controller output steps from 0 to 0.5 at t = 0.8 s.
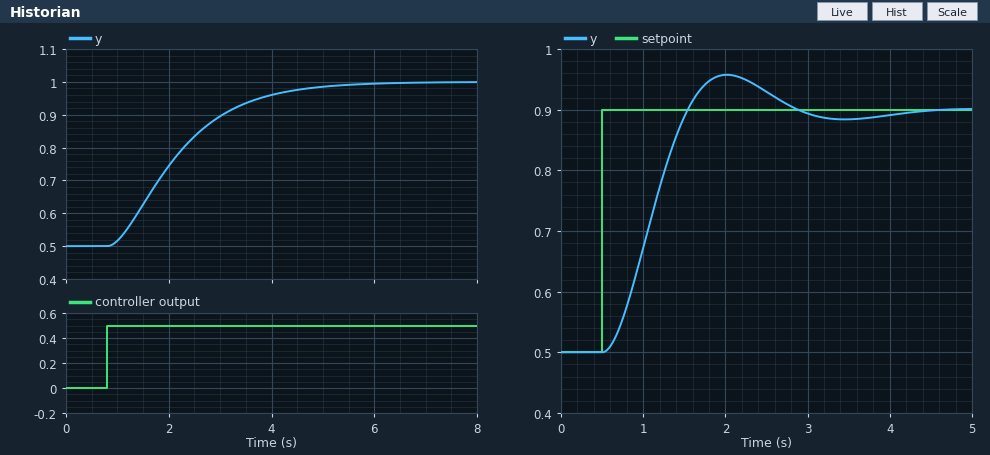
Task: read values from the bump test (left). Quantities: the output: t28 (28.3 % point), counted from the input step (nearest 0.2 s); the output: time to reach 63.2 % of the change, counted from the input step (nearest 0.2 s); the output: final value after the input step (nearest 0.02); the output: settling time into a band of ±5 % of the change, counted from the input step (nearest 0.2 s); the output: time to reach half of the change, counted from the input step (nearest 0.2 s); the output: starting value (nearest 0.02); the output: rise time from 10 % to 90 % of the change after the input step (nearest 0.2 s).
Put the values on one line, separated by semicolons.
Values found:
0.8 s; 1.6 s; 1.00; 3.6 s; 1.2 s; 0.50; 2.6 s
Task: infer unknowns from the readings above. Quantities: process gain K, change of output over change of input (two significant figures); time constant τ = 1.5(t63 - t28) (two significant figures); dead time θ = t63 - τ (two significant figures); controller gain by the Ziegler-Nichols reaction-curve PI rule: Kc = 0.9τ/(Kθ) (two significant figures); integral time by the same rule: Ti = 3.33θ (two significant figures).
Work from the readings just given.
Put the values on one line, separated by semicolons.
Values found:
1.0; 1.2 s; 0.40 s; 2.7; 1.3 s
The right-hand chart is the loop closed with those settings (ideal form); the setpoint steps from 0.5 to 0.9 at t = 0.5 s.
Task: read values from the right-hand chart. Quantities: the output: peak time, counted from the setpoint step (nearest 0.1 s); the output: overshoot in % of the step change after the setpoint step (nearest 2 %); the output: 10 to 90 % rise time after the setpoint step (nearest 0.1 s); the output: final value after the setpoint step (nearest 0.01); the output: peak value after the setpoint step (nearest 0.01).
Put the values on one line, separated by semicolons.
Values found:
1.5 s; 14 %; 0.7 s; 0.90; 0.96
